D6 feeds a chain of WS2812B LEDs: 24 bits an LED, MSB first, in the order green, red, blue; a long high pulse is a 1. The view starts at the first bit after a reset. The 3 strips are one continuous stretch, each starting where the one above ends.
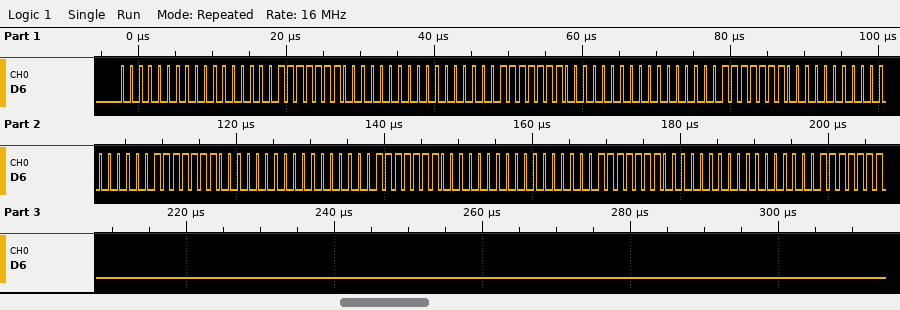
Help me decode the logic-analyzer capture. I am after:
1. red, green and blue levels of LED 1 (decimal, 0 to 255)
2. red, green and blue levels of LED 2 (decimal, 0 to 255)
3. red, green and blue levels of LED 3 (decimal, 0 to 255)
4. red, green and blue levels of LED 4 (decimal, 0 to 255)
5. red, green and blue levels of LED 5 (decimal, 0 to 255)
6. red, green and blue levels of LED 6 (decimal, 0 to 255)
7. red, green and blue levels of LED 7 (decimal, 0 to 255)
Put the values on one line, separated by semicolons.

0, 0, 127; 0, 0, 127; 0, 0, 127; 0, 0, 127; 0, 0, 127; 0, 0, 127; 0, 0, 127
